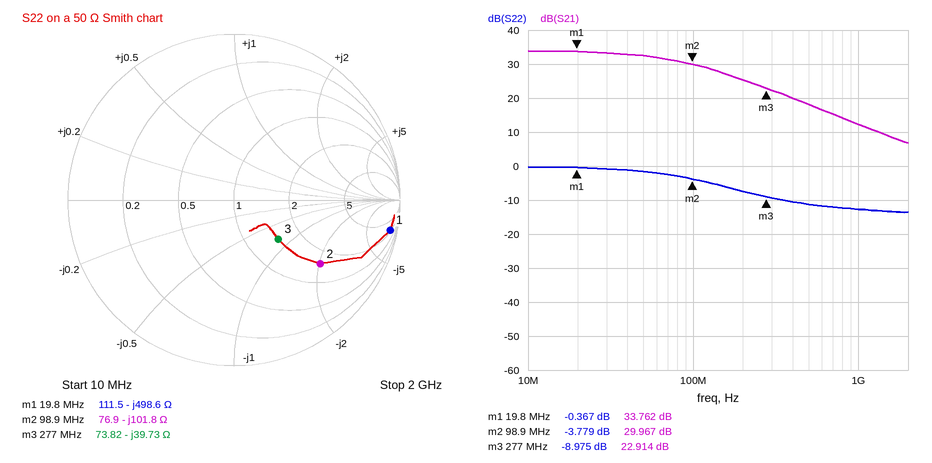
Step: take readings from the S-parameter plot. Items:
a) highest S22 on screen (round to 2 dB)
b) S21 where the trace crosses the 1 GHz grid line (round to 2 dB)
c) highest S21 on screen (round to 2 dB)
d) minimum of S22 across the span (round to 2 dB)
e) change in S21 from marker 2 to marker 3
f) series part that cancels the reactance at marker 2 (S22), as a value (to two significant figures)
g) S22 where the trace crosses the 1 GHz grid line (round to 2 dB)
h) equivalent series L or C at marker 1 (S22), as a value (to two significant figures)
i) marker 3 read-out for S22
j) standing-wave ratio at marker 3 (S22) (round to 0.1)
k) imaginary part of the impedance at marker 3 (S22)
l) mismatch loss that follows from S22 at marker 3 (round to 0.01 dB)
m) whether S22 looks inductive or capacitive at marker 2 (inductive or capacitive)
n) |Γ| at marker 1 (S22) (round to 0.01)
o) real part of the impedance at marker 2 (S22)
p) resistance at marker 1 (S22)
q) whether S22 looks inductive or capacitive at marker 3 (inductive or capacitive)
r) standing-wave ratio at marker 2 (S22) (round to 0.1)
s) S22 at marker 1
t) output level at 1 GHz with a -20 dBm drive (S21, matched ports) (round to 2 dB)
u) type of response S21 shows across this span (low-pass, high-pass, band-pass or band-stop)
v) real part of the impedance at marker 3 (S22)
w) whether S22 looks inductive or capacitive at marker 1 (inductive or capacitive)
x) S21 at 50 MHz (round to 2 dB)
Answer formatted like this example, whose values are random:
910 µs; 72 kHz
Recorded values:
0 dB; 12 dB; 34 dB; -14 dB; -7.053 dB; 160 nH; -12 dB; 16 pF; -8.975 dB; 2.1; -39.73 Ω; 0.59 dB; capacitive; 0.96; 76.9 Ω; 111.5 Ω; capacitive; 4.7; -0.367 dB; -8 dBm; low-pass; 73.82 Ω; capacitive; 32 dB
